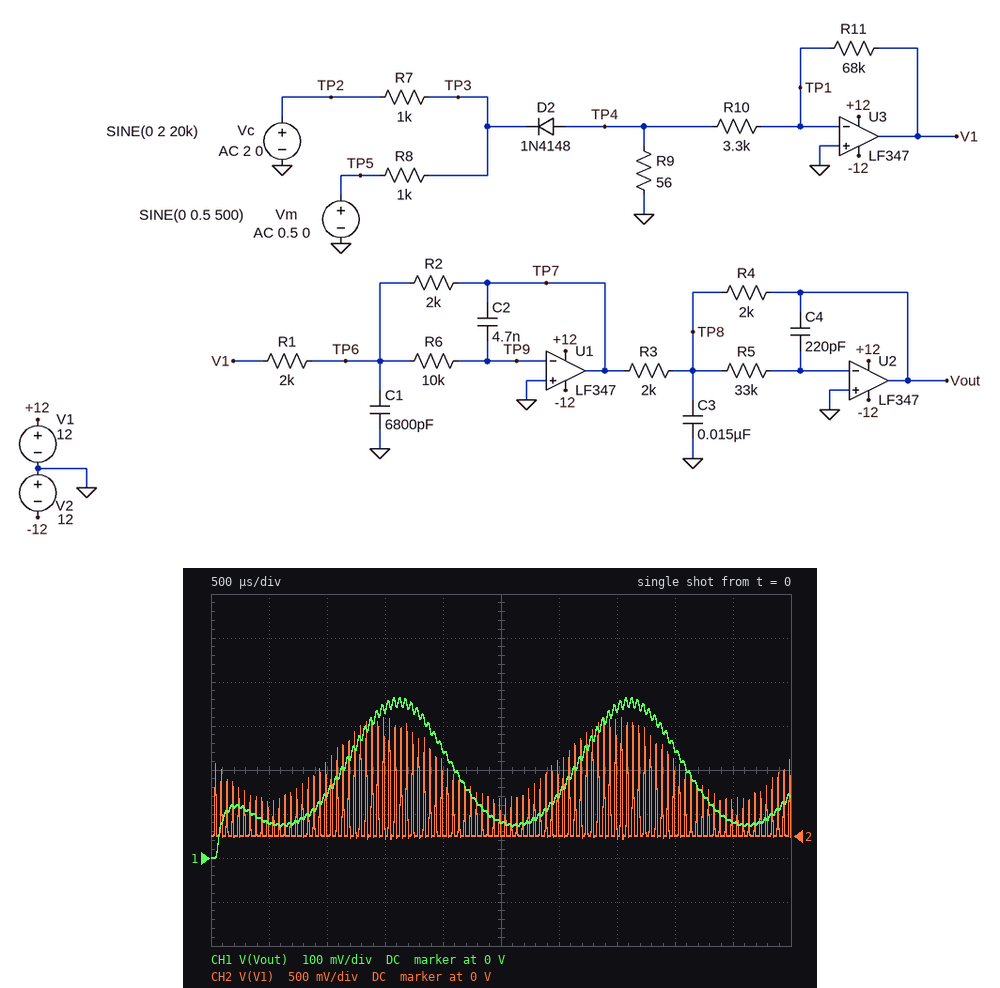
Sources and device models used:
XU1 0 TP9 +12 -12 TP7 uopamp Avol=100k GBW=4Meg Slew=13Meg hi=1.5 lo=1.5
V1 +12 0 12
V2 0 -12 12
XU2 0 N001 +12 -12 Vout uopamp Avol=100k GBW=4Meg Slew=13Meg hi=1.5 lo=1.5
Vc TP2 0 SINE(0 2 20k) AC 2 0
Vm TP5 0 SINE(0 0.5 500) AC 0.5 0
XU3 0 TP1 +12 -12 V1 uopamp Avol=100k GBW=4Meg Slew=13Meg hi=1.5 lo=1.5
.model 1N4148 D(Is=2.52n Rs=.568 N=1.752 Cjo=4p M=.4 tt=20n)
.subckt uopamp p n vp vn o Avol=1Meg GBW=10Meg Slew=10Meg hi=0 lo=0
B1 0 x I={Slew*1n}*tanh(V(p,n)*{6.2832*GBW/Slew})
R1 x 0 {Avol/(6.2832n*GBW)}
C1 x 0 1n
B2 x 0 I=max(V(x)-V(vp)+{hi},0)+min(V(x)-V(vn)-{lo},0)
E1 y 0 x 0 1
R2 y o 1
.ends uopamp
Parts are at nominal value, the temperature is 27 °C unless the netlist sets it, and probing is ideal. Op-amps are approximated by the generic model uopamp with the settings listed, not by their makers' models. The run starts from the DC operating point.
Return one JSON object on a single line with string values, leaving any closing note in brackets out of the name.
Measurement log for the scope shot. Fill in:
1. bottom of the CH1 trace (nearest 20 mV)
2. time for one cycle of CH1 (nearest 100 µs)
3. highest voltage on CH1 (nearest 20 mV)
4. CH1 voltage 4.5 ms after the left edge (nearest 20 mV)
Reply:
{"bottom of the CH1 trace": "0 V", "time for one cycle of CH1": "2.0 ms", "highest voltage on CH1": "360 mV", "CH1 voltage 4.5 ms after the left edge": "80 mV"}
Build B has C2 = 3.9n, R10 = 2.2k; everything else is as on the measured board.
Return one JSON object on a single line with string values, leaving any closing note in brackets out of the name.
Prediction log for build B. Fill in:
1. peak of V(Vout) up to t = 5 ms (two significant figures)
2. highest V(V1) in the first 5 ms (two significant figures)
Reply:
{"peak of V(Vout) up to t = 5 ms": "550 mV", "highest V(V1) in the first 5 ms": "2.0 V"}
